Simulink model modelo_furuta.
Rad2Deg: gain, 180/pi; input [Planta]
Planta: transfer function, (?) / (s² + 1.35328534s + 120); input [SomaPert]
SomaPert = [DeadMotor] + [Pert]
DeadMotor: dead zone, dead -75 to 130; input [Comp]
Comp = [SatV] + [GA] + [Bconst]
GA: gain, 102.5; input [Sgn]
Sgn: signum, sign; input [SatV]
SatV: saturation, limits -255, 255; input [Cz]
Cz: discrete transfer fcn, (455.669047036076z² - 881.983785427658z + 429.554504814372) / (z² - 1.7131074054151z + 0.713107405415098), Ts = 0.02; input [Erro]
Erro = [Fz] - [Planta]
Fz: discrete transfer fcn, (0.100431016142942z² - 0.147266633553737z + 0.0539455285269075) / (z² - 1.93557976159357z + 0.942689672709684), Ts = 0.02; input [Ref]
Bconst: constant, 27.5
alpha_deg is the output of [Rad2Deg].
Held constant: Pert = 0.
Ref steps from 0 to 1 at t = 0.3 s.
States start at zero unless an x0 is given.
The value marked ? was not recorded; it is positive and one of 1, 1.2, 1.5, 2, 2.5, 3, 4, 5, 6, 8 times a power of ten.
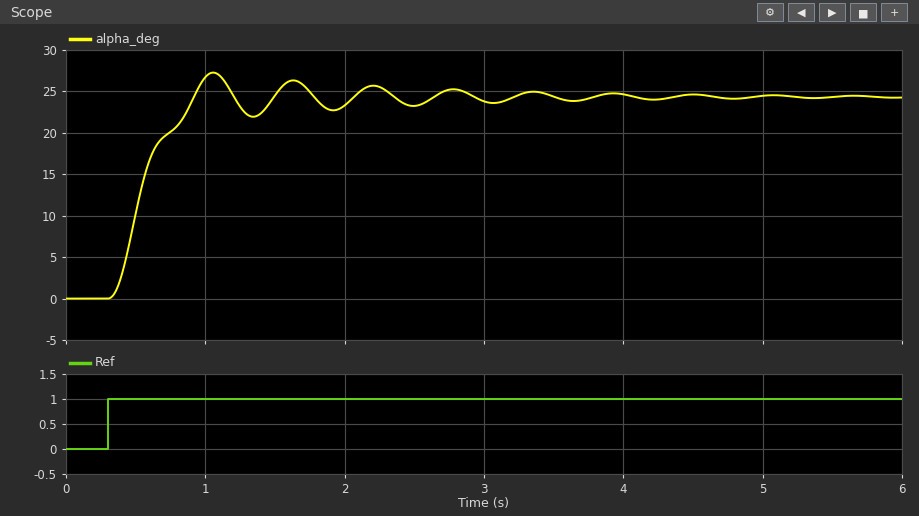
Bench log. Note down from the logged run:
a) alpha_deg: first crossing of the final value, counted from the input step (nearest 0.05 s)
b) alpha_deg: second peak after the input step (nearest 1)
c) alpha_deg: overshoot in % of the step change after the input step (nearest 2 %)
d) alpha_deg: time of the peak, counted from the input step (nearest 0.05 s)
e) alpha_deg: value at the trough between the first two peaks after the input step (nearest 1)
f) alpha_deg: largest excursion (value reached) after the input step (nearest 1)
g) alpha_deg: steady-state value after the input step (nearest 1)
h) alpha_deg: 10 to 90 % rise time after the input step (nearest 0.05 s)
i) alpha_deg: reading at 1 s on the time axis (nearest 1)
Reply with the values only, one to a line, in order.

0.60 s
26
12 %
0.75 s
22
27
24
0.45 s
27
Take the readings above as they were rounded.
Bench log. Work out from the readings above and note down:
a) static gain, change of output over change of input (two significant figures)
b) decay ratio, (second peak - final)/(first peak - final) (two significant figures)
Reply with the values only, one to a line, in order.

24
0.67
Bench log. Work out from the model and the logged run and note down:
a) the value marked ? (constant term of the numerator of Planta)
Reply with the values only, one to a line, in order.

0.2
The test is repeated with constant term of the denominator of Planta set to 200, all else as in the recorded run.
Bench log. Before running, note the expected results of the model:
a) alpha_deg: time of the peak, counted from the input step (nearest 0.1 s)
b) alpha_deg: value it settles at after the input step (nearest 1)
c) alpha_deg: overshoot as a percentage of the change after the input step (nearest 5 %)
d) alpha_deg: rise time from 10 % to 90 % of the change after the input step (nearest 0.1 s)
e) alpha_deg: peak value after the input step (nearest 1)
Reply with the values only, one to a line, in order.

0.6 s
15
15 %
0.4 s
17
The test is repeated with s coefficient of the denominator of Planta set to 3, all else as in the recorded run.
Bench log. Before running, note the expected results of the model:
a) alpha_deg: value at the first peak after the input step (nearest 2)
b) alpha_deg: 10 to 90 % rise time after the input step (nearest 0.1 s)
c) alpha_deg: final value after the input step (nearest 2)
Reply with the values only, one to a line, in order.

26
0.4 s
24
